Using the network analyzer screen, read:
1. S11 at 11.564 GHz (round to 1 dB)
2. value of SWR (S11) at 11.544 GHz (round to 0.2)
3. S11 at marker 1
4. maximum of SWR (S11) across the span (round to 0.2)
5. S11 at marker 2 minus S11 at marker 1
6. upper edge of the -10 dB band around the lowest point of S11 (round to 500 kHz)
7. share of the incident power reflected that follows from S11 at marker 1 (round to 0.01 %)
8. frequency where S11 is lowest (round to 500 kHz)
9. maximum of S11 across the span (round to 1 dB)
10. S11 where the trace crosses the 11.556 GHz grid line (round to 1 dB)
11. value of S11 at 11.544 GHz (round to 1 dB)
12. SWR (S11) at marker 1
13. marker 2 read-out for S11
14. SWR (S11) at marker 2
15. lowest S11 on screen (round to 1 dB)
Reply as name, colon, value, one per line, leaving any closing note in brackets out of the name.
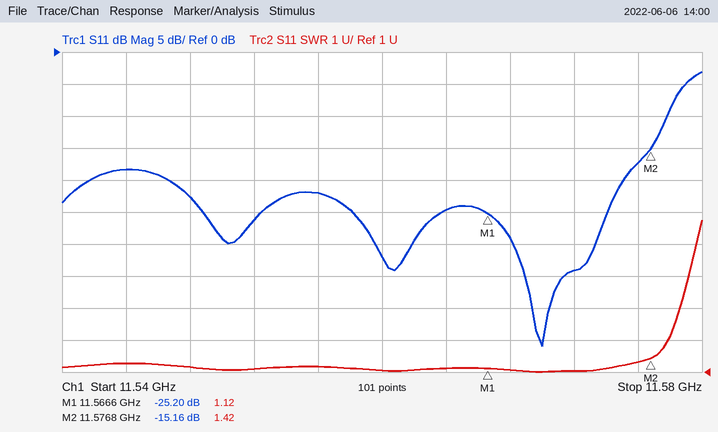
S11 at 11.564 GHz: -25 dB
value of SWR (S11) at 11.544 GHz: 1.2
S11 at marker 1: -25.20 dB
maximum of SWR (S11) across the span: 5.8
S11 at marker 2 minus S11 at marker 1: 10.04 dB
upper edge of the -10 dB band around the lowest point of S11: 11.5780 GHz
share of the incident power reflected that follows from S11 at marker 1: 0.30 %
frequency where S11 is lowest: 11.5700 GHz
maximum of S11 across the span: -3 dB
S11 where the trace crosses the 11.556 GHz grid line: -22 dB
value of S11 at 11.544 GHz: -18 dB
SWR (S11) at marker 1: 1.12
marker 2 read-out for S11: -15.16 dB
SWR (S11) at marker 2: 1.42
lowest S11 on screen: -46 dB
